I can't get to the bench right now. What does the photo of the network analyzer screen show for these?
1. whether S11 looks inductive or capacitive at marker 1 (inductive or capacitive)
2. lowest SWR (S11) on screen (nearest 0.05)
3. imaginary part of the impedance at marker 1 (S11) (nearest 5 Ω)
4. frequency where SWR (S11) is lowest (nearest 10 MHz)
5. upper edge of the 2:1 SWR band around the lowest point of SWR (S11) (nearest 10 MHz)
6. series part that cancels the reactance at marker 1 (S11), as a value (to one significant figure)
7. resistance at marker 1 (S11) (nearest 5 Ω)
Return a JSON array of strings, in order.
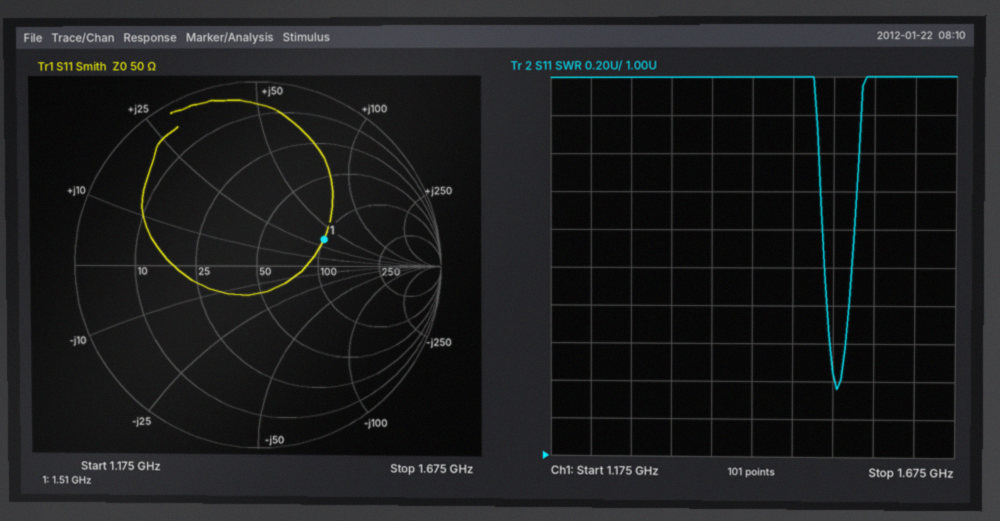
["inductive", "1.35", "+35 Ω", "1.53 GHz", "1.55 GHz", "3 pF", "100 Ω"]
